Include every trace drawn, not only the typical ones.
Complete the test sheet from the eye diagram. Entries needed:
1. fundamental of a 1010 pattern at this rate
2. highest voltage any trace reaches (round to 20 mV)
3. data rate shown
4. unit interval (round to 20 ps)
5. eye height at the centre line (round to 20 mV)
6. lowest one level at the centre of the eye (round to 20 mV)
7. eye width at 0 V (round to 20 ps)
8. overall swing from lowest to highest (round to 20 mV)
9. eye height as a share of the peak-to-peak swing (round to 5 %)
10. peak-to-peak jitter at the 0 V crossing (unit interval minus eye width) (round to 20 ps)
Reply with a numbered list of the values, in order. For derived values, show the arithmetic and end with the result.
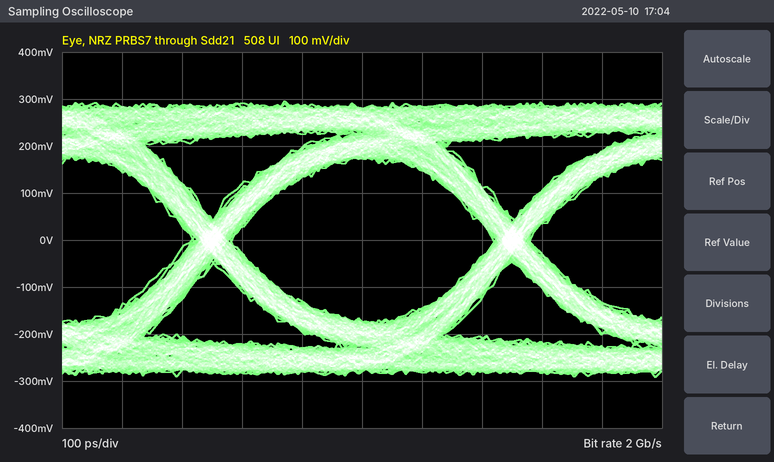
1. 1 GHz
2. 300 mV
3. 2 Gb/s
4. 500 ps
5. 340 mV
6. 180 mV
7. 440 ps
8. 580 mV
9. 340 mV / 580 mV ≈ 58.6 %, so 60 % to the nearest 5 %
10. 60 ps
